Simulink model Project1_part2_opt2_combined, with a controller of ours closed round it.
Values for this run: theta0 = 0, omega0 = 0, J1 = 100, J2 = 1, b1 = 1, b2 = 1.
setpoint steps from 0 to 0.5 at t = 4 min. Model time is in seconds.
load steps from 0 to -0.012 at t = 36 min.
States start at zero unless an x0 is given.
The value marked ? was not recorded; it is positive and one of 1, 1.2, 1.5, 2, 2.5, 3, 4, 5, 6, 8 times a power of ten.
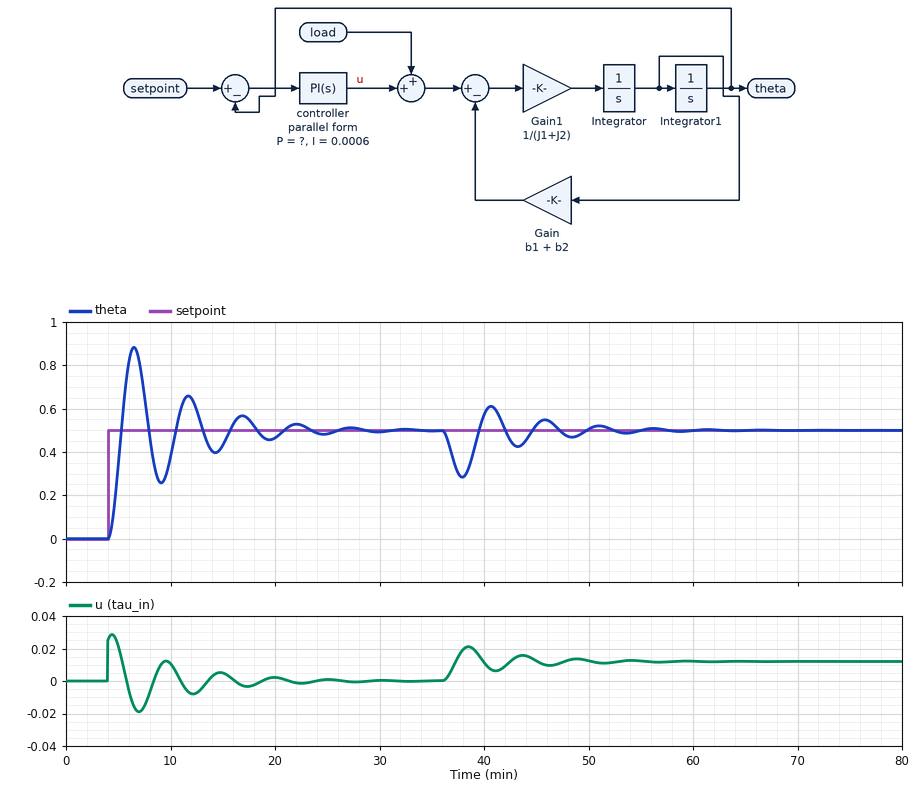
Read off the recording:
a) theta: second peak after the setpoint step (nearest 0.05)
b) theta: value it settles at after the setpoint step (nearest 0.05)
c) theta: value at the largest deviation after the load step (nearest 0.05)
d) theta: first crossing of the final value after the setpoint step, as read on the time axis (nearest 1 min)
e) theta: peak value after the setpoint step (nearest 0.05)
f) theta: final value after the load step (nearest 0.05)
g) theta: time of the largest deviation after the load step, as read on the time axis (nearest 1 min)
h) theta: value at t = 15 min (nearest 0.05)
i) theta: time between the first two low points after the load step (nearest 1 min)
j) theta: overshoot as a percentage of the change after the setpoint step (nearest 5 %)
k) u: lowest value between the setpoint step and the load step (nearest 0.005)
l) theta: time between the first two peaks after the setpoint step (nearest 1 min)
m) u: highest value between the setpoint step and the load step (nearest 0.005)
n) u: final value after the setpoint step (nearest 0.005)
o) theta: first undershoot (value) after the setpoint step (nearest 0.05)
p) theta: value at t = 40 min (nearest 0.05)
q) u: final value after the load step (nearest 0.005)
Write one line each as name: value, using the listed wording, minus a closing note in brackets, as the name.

theta: second peak after the setpoint step: 0.65
theta: value it settles at after the setpoint step: 0.50
theta: value at the largest deviation after the load step: 0.30
theta: first crossing of the final value after the setpoint step, as read on the time axis: 5 min
theta: peak value after the setpoint step: 0.90
theta: final value after the load step: 0.50
theta: time of the largest deviation after the load step, as read on the time axis: 38 min
theta: value at t = 15 min: 0.45
theta: time between the first two low points after the load step: 5 min
theta: overshoot as a percentage of the change after the setpoint step: 75 %
u: lowest value between the setpoint step and the load step: -0.020
theta: time between the first two peaks after the setpoint step: 5 min
u: highest value between the setpoint step and the load step: 0.030
u: final value after the setpoint step: 0.000
theta: first undershoot (value) after the setpoint step: 0.25
theta: value at t = 40 min: 0.55
u: final value after the load step: 0.010
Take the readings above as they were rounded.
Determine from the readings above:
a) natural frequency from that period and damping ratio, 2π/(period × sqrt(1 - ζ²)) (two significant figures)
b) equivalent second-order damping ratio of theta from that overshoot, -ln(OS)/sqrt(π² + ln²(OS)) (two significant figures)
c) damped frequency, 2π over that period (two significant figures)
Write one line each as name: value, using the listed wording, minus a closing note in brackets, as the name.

natural frequency from that period and damping ratio, 2π/(period × sqrt(1 - ζ²)): 1.3 rad/min
equivalent second-order damping ratio of theta from that overshoot, -ln(OS)/sqrt(π² + ln²(OS)): 0.091
damped frequency, 2π over that period: 1.3 rad/min
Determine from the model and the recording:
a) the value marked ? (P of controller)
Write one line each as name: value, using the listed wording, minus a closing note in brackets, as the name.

the value marked ?: 0.05
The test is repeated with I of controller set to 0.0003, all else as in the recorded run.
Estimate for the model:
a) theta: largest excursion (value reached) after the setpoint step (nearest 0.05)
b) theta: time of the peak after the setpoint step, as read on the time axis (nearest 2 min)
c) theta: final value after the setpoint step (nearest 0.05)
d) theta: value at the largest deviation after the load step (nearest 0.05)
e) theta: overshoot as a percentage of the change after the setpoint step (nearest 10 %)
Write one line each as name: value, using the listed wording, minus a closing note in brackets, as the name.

theta: largest excursion (value reached) after the setpoint step: 0.75
theta: time of the peak after the setpoint step, as read on the time axis: 6 min
theta: final value after the setpoint step: 0.50
theta: value at the largest deviation after the load step: 0.25
theta: overshoot as a percentage of the change after the setpoint step: 50 %
